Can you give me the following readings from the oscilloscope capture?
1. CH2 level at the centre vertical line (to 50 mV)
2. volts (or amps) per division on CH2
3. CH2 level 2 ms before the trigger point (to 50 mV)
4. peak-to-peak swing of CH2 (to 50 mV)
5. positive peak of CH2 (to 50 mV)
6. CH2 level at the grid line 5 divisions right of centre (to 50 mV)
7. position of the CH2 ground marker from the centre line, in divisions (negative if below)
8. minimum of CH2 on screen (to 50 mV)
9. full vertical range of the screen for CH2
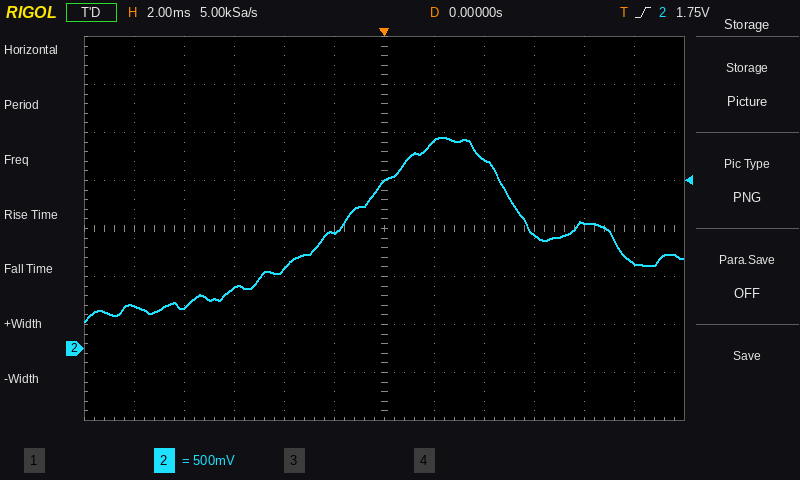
1.75 V
500 mV
1.20 V
1.90 V
2.20 V
900 mV
-2.5 div
300 mV
4 V
